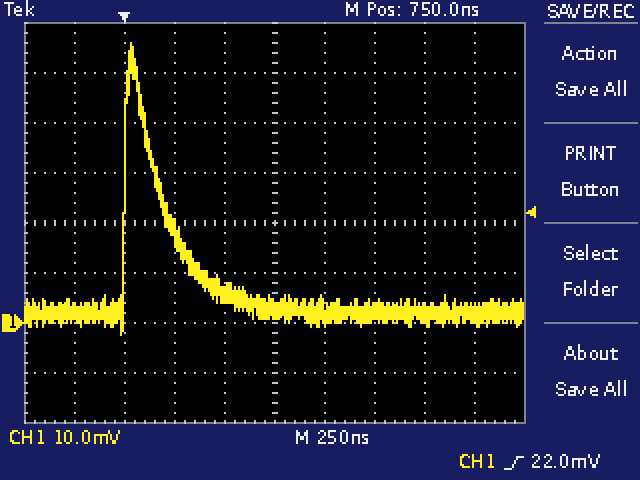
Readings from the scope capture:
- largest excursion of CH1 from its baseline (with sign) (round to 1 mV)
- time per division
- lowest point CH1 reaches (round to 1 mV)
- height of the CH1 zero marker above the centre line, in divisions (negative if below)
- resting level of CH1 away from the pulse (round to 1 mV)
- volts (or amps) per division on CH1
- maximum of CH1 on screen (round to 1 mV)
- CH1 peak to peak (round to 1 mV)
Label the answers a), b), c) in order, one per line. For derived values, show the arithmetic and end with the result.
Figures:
a) 56 mV − (2 mV) = +54 mV
b) 250 ns
c) -2 mV
d) -2.0 div
e) 2 mV
f) 10 mV
g) 56 mV
h) 56 mV − (-2 mV) = 58 mV
